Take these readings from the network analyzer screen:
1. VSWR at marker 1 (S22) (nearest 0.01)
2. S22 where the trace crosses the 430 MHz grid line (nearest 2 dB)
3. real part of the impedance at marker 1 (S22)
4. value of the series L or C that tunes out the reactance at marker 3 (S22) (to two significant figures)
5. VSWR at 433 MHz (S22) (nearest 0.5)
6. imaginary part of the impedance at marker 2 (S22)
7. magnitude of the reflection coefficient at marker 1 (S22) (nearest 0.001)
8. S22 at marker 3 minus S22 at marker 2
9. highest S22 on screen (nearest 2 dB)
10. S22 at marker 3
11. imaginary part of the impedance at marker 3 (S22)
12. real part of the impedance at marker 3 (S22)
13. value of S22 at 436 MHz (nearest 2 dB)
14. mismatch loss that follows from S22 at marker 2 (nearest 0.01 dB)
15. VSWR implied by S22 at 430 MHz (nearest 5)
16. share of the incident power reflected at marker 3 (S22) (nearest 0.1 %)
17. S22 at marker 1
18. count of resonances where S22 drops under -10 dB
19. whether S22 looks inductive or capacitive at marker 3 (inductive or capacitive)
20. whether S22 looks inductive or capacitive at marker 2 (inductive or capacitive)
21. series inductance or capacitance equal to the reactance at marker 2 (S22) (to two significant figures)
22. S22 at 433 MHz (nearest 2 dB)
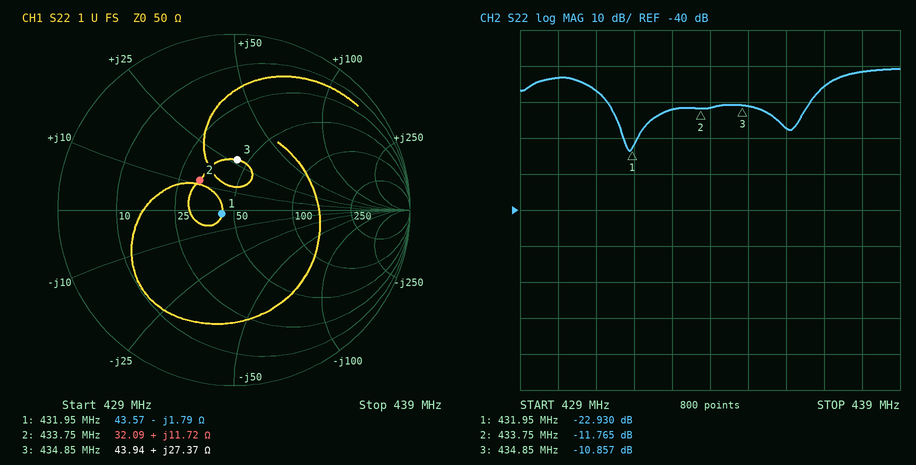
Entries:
1.15
-4 dB
43.57 Ω
13 pF
1.5
+11.72 Ω
0.071
0.908 dB
0 dB
-10.857 dB
+27.37 Ω
43.94 Ω
-18 dB
0.30 dB
5
8.2 %
-22.930 dB
2
inductive
inductive
4.3 nH
-12 dB
